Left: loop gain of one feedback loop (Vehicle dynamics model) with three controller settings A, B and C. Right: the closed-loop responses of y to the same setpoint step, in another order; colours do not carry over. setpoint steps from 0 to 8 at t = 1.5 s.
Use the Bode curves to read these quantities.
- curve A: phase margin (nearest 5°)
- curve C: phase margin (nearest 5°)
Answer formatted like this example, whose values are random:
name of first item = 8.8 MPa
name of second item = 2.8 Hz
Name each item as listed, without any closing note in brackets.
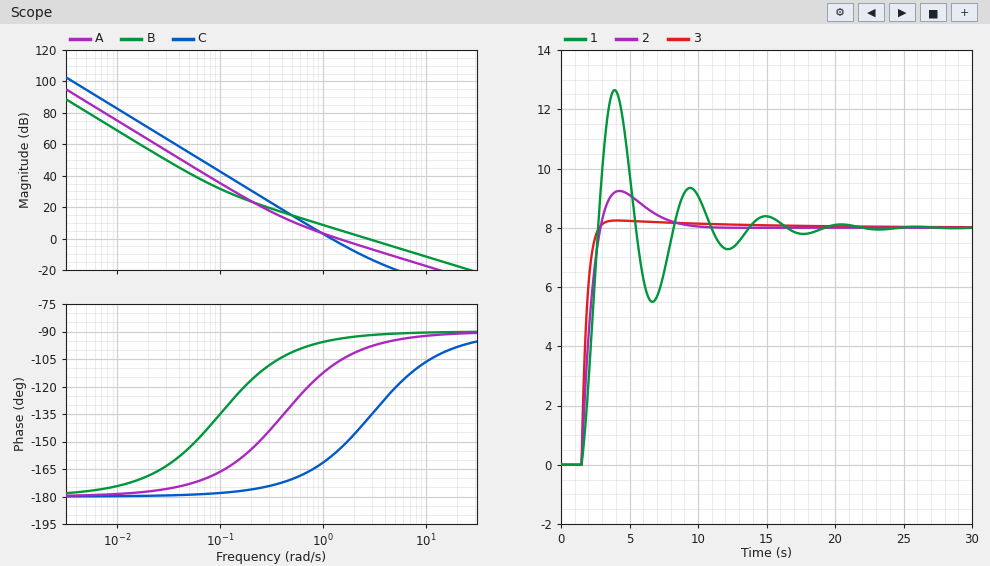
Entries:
curve A: phase margin = 75°
curve C: phase margin = 20°
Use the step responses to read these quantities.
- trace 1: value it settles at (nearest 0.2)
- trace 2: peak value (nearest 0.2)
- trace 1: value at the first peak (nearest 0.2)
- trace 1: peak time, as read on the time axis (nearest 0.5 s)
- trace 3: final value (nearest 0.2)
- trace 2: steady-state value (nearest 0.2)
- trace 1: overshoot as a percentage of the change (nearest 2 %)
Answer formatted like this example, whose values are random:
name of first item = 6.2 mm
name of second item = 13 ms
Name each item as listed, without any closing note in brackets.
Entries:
trace 1: value it settles at = 8.0
trace 2: peak value = 9.2
trace 1: value at the first peak = 12.6
trace 1: peak time, as read on the time axis = 4.0 s
trace 3: final value = 8.0
trace 2: steady-state value = 8.0
trace 1: overshoot as a percentage of the change = 58 %
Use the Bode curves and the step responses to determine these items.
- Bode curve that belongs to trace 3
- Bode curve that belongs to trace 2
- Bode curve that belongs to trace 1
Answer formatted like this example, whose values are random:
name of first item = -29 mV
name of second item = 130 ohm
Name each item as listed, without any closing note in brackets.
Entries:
Bode curve that belongs to trace 3 = B
Bode curve that belongs to trace 2 = A
Bode curve that belongs to trace 1 = C
